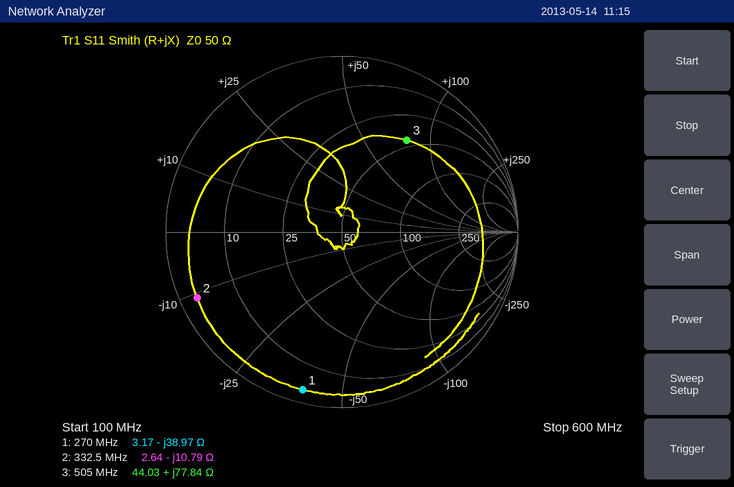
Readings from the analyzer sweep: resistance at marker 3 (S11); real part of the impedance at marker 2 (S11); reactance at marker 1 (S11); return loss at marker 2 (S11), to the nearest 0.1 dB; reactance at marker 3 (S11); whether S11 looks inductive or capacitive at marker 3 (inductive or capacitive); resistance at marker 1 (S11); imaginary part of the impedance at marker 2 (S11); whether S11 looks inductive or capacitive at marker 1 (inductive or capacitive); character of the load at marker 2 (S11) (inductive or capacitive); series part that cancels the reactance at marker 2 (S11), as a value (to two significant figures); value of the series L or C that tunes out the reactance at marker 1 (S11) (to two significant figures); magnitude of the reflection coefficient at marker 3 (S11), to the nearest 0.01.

44.03 Ω
2.64 Ω
-38.97 Ω
0.9 dB
+77.84 Ω
inductive
3.17 Ω
-10.79 Ω
capacitive
capacitive
5.2 nH
23 nH
0.64
